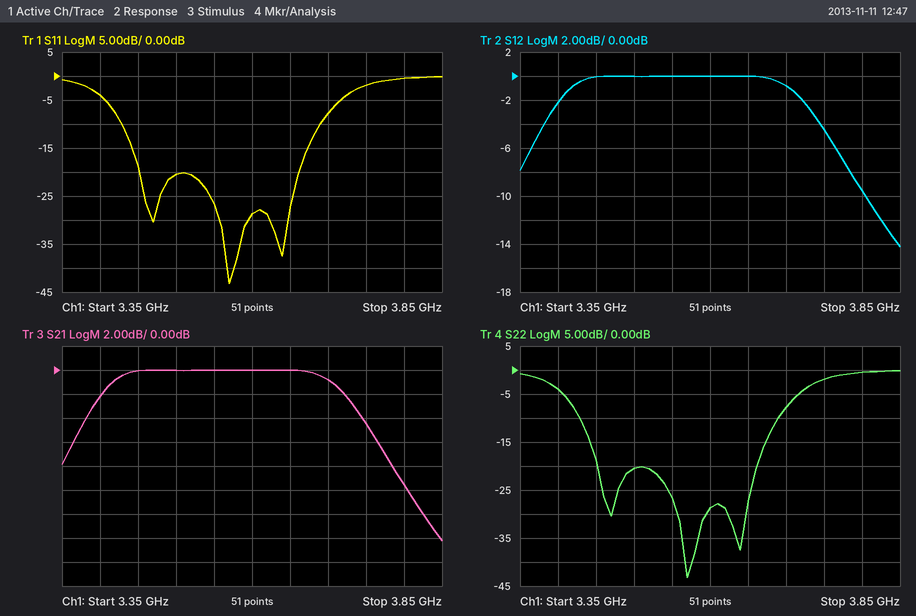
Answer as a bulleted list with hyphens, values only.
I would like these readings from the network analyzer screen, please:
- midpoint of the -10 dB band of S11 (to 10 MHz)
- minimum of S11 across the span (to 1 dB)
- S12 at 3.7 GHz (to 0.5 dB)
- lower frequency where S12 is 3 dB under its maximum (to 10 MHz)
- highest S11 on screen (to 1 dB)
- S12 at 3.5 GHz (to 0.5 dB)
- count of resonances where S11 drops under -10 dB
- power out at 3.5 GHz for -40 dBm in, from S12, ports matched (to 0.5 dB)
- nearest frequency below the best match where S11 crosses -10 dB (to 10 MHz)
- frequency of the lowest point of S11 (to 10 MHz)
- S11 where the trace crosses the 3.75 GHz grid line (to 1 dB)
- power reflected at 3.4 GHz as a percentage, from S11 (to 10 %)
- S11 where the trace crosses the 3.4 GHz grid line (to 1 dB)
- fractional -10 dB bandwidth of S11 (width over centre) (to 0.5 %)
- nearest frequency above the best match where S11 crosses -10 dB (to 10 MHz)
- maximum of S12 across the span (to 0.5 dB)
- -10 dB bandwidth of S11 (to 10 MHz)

- 3.56 GHz
- -43 dB
- -1.0 dB
- 3.39 GHz
- 0 dB
- 0.0 dB
- 3
- -40.0 dBm
- 3.43 GHz
- 3.57 GHz
- -2 dB
- 40 %
- -4 dB
- 7.5 %
- 3.69 GHz
- 0.0 dB
- 260 MHz
